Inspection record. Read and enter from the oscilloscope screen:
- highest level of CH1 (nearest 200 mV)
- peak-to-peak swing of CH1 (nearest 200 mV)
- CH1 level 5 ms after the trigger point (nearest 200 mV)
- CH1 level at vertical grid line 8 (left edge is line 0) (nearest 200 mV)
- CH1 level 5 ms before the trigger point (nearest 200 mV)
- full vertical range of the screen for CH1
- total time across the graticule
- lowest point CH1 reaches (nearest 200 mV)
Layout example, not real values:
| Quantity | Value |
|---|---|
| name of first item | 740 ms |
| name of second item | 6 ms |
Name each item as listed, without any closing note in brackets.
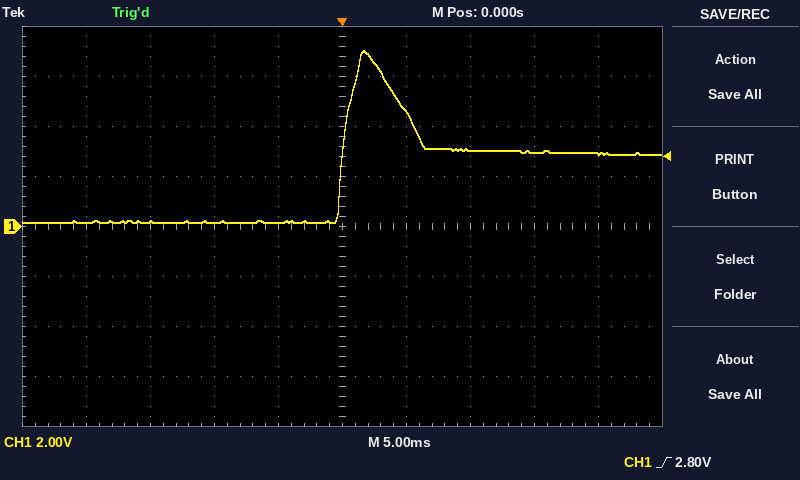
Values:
| Quantity | Value |
|---|---|
| highest level of CH1 | 7.0 V |
| peak-to-peak swing of CH1 | 6.8 V |
| CH1 level 5 ms after the trigger point | 4.6 V |
| CH1 level at vertical grid line 8 (left edge is line 0) | 3.0 V |
| CH1 level 5 ms before the trigger point | 200 mV |
| full vertical range of the screen for CH1 | 16 V |
| total time across the graticule | 50 ms |
| lowest point CH1 reaches | 200 mV |
